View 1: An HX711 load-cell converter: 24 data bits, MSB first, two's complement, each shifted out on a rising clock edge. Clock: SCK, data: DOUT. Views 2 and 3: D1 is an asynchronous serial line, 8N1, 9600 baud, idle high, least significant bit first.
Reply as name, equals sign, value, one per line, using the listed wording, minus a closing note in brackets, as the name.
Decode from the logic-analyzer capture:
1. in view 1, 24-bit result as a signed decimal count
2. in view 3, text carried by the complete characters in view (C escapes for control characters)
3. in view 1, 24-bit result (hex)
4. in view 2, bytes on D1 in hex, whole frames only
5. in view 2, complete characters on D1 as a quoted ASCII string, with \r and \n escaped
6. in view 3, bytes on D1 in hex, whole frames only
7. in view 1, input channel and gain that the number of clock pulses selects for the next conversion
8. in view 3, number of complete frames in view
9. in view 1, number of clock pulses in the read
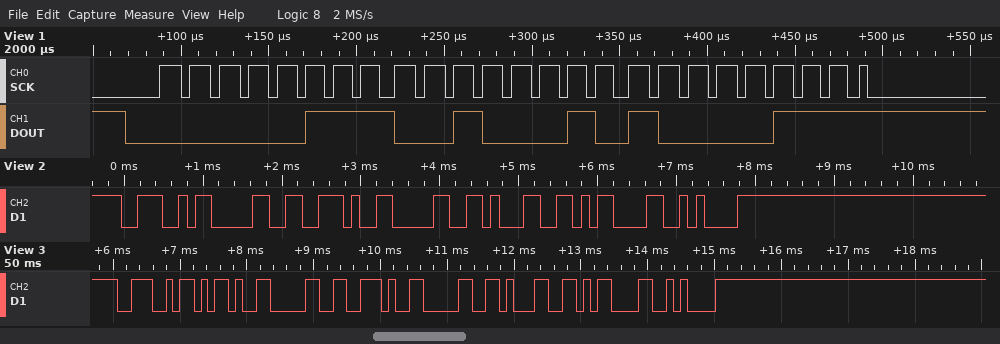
in view 1, 24-bit result as a signed decimal count = 467591
in view 3, text carried by the complete characters in view = "N-0.01\r\n"
in view 1, 24-bit result = 0x072287
in view 2, bytes on D1 in hex, whole frames only = 4E 30 2E 30 31 0D 0A
in view 2, complete characters on D1 as a quoted ASCII string, with \r and \n escaped = "N0.01\r\n"
in view 3, bytes on D1 in hex, whole frames only = 4E 2D 30 2E 30 31 0D 0A
in view 1, input channel and gain that the number of clock pulses selects for the next conversion = channel A, gain 128
in view 3, number of complete frames in view = 8
in view 1, number of clock pulses in the read = 25
